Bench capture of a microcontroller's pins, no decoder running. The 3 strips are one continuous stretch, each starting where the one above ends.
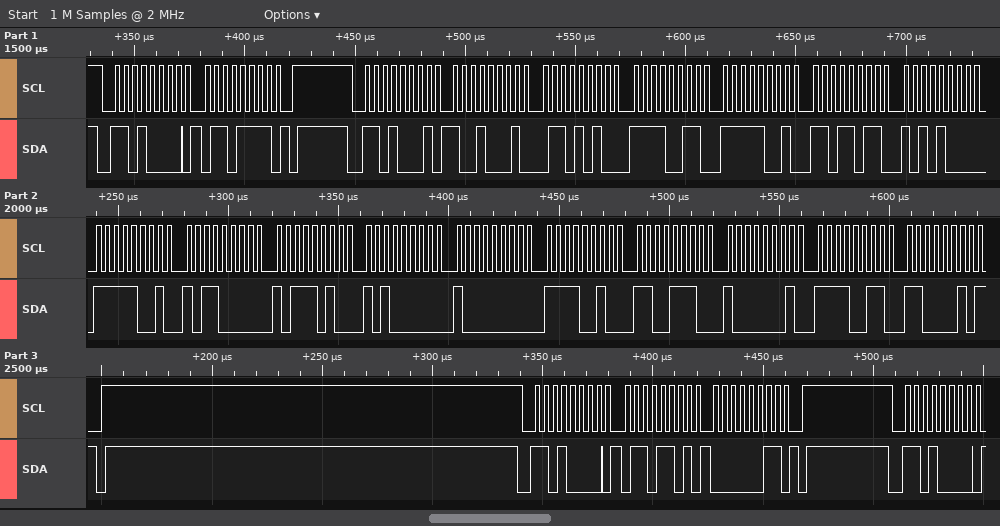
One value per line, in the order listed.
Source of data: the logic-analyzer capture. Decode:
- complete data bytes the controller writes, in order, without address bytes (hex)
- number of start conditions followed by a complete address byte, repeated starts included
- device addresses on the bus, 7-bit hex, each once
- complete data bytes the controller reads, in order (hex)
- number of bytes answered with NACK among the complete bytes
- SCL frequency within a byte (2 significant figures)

6F 6D 03
4
0x68
91 6A F3 F9 DB A8 F9 B0 BA A0 80 F2 CE 81 F3 C2
1
250 kHz
